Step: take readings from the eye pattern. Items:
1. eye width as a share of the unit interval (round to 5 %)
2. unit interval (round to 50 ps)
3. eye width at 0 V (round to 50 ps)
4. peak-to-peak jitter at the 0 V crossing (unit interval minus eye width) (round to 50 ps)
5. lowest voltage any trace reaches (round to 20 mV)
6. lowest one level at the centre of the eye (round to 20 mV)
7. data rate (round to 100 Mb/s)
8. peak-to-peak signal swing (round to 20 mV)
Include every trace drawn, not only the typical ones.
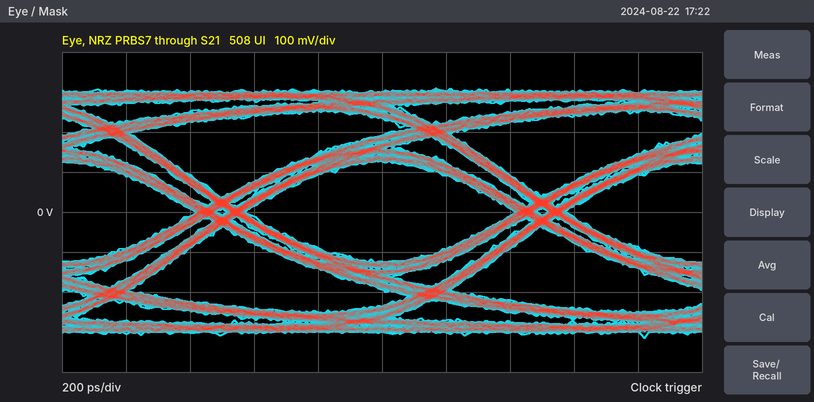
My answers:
85 %
1.00 ns
850 ps
150 ps
-320 mV
120 mV
1.0 Gb/s
620 mV
